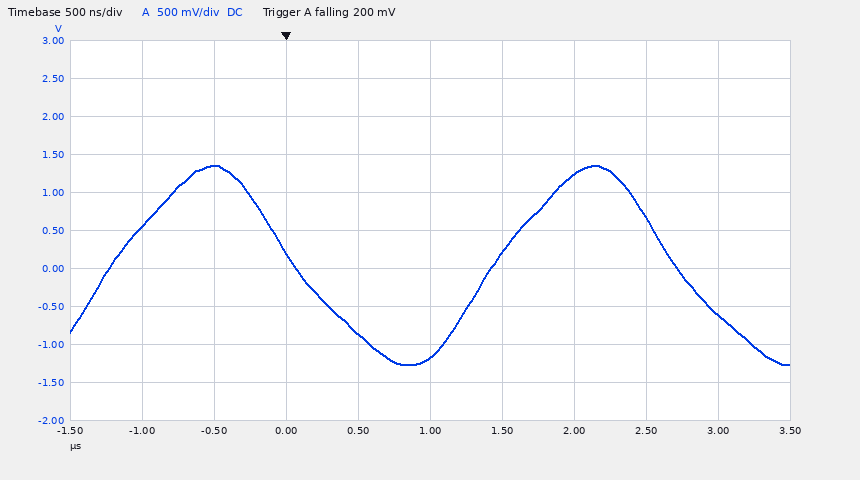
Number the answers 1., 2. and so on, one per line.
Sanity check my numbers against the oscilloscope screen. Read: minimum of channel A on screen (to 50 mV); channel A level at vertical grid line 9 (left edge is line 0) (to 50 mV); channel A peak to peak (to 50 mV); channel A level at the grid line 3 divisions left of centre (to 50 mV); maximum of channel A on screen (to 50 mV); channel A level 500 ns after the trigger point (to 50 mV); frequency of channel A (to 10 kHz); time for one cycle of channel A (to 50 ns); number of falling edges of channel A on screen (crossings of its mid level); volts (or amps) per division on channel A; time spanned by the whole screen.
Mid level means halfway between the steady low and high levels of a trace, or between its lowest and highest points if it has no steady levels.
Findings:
1. -1.25 V
2. -600 mV
3. 2.60 V
4. 1.35 V
5. 1.35 V
6. -850 mV
7. 380 kHz
8. 2.65 µs
9. 2
10. 500 mV
11. 5 µs
